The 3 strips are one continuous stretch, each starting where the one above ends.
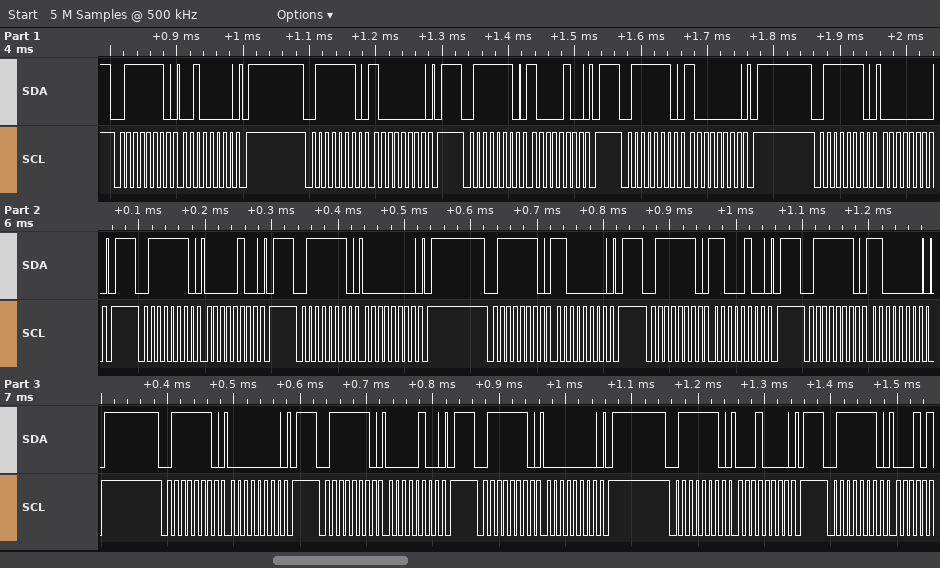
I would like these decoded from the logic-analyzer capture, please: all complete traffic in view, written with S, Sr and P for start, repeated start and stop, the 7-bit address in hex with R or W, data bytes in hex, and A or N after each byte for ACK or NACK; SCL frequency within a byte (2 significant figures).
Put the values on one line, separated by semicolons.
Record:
S 3FW A 20 A P S 3FW A 80 A P S 3FW A 84 A P S 3FW A 80 A P S 3FW A 00 A P S 3FW A 04 A P S 3FW A 00 A P S 3FW A C0 A P S 3FW A C4 A P S 3FW A C0 A P S 3FW A 00 A P S 3FW A 04 A P S 3FW A 00 A P S 3FW A 10 A P S 3FW A; 100 kHz
